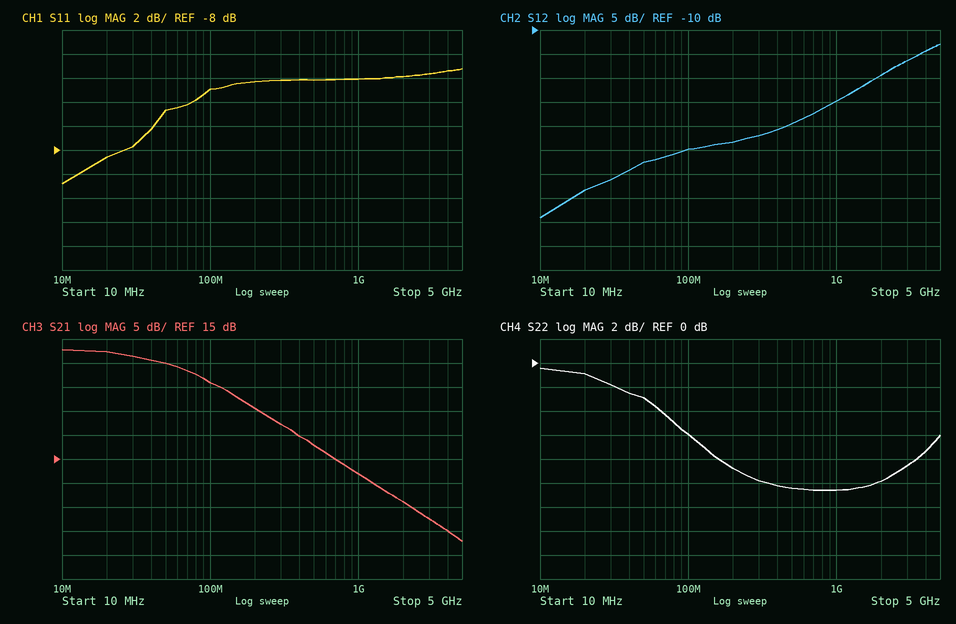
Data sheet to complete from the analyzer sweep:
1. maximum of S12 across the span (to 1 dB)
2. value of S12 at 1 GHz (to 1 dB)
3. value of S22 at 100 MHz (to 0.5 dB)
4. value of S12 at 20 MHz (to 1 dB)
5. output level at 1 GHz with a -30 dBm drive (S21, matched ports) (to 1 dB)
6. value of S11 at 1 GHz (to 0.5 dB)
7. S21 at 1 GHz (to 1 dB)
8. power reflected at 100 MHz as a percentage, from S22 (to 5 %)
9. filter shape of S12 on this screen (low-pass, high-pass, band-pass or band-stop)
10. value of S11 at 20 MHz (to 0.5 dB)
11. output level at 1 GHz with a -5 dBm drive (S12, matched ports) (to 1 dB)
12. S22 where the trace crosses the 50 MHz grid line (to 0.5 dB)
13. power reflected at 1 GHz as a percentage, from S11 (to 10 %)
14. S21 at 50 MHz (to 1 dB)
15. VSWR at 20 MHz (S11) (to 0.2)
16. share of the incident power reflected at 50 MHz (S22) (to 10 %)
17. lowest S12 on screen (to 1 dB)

-13 dB
-25 dB
-6.0 dB
-43 dB
-18 dBm
-2.0 dB
12 dB
25 %
high-pass
-8.5 dB
-30 dBm
-3.0 dB
60 %
35 dB
2.2
50 %
-49 dB
